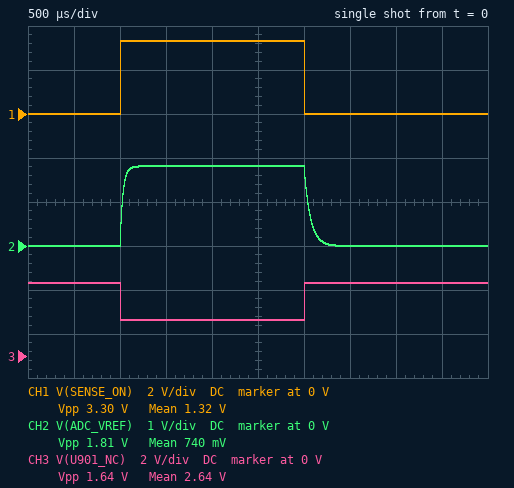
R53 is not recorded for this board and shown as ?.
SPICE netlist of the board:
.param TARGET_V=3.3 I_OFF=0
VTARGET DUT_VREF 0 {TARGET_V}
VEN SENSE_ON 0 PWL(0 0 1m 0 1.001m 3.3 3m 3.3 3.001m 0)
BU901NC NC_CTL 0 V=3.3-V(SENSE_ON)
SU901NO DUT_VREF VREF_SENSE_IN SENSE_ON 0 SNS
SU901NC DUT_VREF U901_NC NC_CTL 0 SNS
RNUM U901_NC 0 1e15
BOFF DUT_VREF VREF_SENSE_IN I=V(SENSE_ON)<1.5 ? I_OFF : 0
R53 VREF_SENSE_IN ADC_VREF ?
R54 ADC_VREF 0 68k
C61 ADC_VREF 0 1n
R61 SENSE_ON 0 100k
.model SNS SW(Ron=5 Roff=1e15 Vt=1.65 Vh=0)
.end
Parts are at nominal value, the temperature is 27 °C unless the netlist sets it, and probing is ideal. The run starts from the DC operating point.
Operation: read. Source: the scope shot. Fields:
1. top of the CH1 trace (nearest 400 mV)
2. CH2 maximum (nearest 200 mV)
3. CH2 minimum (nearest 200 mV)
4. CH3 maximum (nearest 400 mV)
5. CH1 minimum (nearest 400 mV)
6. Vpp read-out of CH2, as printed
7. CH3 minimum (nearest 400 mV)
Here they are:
3.2 V
1.8 V
0 V
3.2 V
0 V
1.81 V
1.6 V
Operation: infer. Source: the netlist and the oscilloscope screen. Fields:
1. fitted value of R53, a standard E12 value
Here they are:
56 kΩ
